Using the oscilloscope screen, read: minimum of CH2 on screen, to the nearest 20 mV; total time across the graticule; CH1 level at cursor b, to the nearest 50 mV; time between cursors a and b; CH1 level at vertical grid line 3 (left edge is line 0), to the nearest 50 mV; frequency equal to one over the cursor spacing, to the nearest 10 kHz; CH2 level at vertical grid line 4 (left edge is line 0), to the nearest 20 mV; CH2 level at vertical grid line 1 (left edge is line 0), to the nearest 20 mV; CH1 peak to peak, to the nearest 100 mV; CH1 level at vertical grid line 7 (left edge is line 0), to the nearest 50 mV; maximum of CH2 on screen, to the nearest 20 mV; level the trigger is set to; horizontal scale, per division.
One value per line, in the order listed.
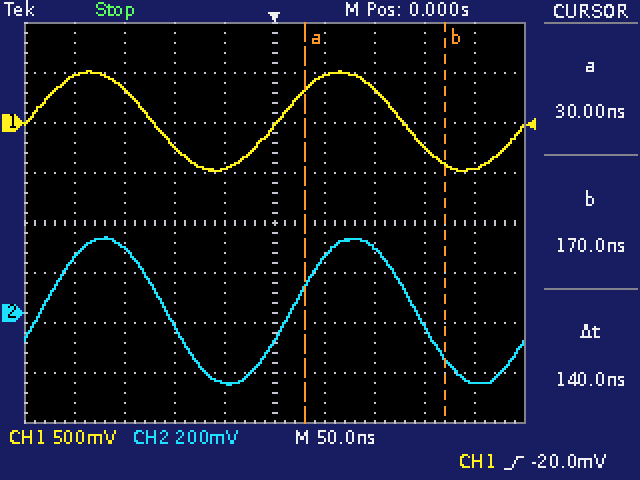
-280 mV
500 ns
-400 mV
140 ns
-250 mV
7.14 MHz
-280 mV
220 mV
1.00 V
350 mV
300 mV
-20.0 mV
50 ns
